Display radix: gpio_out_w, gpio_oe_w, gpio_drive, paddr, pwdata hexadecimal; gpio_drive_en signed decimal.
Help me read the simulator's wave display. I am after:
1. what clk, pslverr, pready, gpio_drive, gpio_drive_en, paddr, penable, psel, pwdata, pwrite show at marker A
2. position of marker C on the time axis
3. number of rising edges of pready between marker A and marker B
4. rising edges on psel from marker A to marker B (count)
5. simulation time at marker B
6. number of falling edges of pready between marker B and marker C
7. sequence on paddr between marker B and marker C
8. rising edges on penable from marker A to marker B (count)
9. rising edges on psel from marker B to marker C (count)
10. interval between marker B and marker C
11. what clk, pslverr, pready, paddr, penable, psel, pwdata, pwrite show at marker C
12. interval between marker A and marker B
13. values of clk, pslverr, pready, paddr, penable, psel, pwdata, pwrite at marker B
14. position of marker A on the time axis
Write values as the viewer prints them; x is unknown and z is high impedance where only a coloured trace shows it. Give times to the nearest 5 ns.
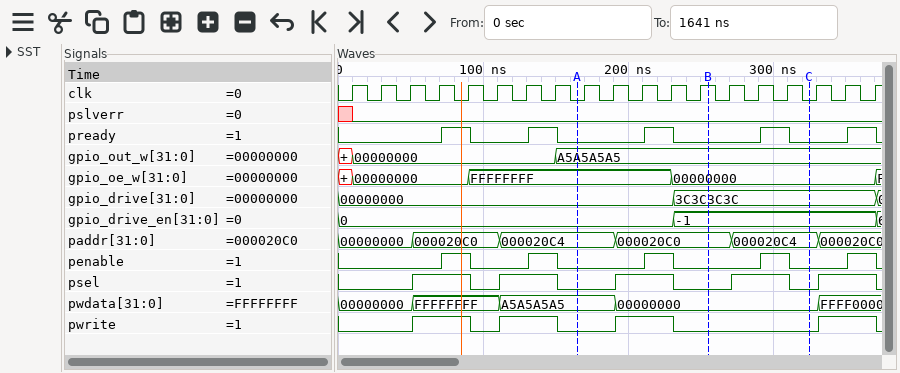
clk=0, pslverr=0, pready=0, gpio_drive=00000000, gpio_drive_en=0, paddr=000020C4, penable=0, psel=0, pwdata=A5A5A5A5, pwrite=0
325 ns
1
1
255 ns
1
000020C0, 000020C4
1
1
70 ns
clk=0, pslverr=0, pready=0, paddr=000020C4, penable=0, psel=0, pwdata=00000000, pwrite=0
90 ns
clk=1, pslverr=0, pready=0, paddr=000020C0, penable=0, psel=0, pwdata=00000000, pwrite=0
165 ns
